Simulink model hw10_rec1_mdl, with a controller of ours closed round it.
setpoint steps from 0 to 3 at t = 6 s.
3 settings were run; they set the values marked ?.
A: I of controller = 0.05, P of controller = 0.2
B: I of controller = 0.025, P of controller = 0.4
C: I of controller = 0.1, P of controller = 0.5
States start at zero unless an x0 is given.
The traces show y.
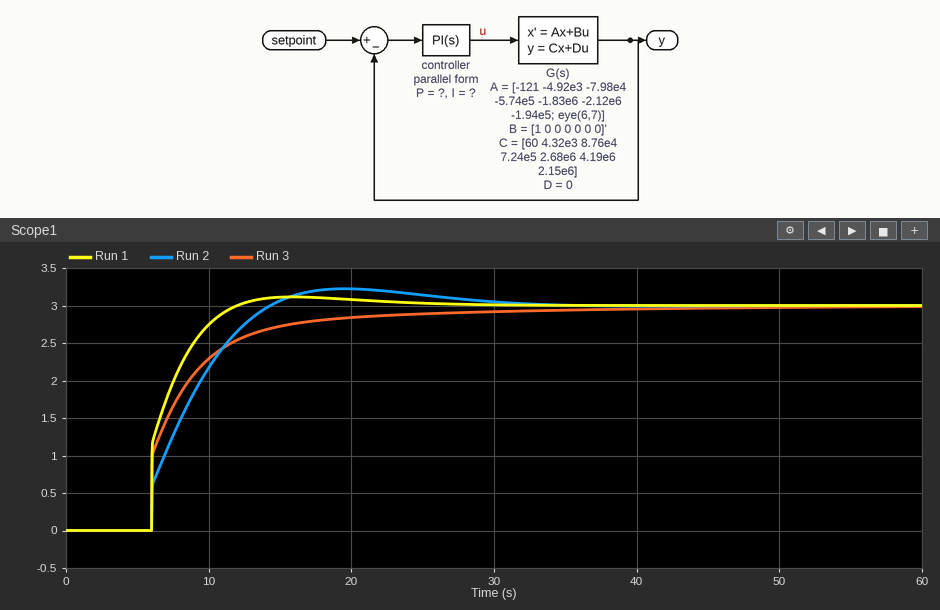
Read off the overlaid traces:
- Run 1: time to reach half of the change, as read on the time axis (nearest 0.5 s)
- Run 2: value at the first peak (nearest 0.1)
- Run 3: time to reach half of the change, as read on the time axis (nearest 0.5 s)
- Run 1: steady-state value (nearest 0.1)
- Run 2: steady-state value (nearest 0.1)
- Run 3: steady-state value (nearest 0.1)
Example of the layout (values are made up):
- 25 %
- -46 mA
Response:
- 6.5 s
- 3.2
- 7.0 s
- 3.0
- 3.0
- 3.0
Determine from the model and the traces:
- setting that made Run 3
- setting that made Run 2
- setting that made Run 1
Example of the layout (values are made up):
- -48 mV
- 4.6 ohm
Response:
- B
- A
- C
